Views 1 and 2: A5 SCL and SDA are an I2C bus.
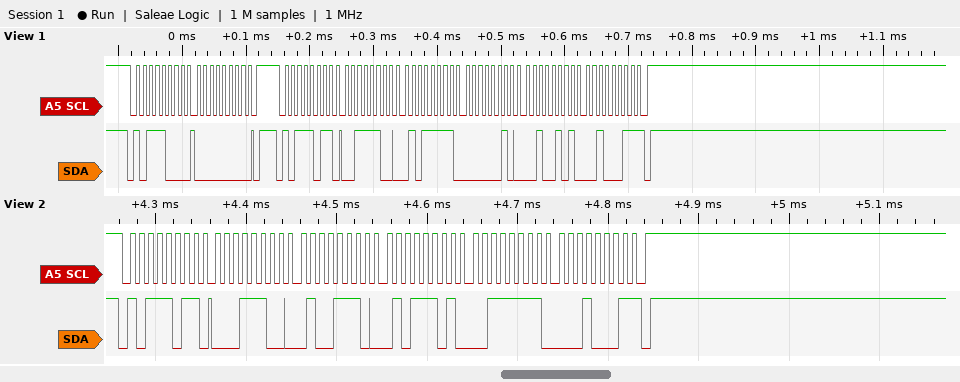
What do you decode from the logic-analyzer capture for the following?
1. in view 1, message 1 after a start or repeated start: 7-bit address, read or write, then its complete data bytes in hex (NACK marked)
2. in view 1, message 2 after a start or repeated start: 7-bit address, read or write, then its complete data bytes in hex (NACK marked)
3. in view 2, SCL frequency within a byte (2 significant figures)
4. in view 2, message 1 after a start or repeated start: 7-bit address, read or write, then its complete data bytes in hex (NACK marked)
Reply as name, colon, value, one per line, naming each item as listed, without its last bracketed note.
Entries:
in view 1, message 1 after a start or repeated start: 7-bit address, read or write, then its complete data bytes in hex: 0x5C write: 00
in view 1, message 2 after a start or repeated start: 7-bit address, read or write, then its complete data bytes in hex: 0x5D read: 3C 5F 02 25 23 NACK
in view 2, SCL frequency within a byte: 100 kHz
in view 2, message 1 after a start or repeated start: 7-bit address, read or write, then its complete data bytes in hex: 0x5D read: 1C 4E 5D 3F 11 NACK
